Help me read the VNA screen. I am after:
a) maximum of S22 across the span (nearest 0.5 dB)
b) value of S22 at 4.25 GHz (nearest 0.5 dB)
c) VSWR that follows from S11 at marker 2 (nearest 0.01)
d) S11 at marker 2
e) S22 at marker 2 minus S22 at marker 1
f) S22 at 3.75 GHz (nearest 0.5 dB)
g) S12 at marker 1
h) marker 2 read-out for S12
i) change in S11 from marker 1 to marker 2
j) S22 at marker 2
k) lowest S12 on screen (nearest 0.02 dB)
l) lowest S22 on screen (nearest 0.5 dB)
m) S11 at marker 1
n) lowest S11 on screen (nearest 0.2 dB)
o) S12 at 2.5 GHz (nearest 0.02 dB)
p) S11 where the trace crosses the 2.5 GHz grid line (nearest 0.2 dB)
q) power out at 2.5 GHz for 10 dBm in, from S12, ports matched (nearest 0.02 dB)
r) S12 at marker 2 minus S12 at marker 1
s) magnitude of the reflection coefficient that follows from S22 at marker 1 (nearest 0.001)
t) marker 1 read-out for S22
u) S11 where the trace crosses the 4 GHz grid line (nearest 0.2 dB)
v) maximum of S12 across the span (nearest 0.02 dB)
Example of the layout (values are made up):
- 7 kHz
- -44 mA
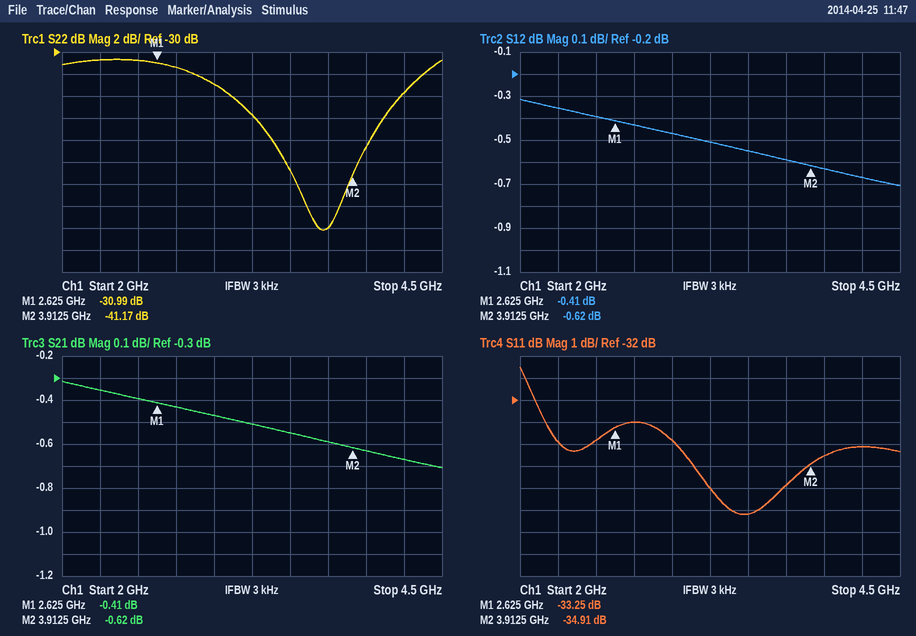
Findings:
- -30.5 dB
- -33.5 dB
- 1.04
- -34.91 dB
- -10.18 dB
- -46.0 dB
- -0.41 dB
- -0.62 dB
- -1.66 dB
- -41.17 dB
- -0.70 dB
- -46.0 dB
- -33.25 dB
- -37.2 dB
- -0.40 dB
- -33.8 dB
- 9.60 dBm
- -0.21 dB
- 0.028
- -30.99 dB
- -34.6 dB
- -0.32 dB
